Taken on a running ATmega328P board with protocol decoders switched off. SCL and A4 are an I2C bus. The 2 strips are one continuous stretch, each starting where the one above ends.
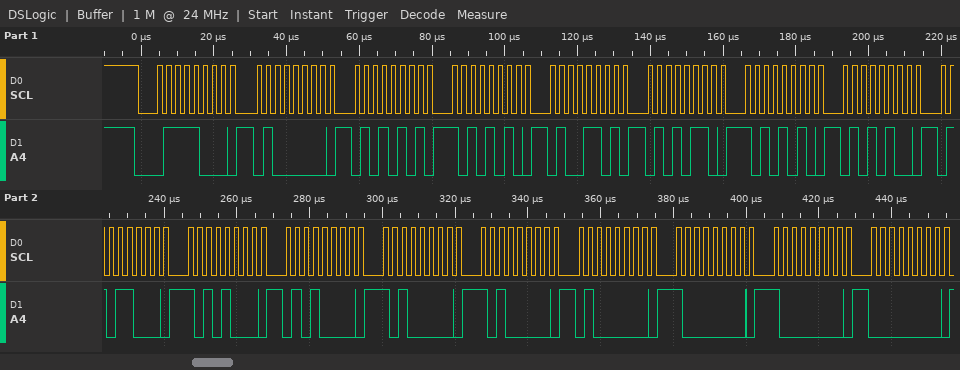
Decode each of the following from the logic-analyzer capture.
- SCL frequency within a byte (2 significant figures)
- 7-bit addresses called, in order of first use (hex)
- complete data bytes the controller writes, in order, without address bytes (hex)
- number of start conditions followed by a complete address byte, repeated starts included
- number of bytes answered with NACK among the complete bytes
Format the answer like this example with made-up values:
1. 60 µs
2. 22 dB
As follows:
1. 400 kHz
2. 0x3C
3. 40 55 AA 4D 56 AA 54 58 A8 50 A0 A0 40 80 80 00
4. 1
5. 0
